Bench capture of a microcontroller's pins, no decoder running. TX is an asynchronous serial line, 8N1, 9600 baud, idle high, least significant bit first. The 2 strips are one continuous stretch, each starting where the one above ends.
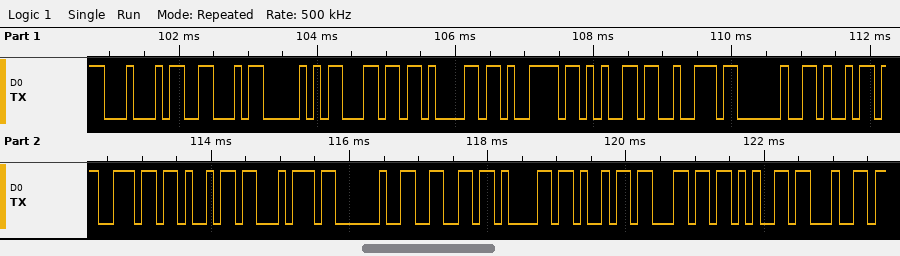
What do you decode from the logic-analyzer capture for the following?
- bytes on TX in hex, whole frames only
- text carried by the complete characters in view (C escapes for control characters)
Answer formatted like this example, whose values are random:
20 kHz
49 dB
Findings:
44 46 50 6C 61 79 65 72 20 69 6E 69 74 20 66 61 69 6C 65 64
"DFPlayer init failed"
